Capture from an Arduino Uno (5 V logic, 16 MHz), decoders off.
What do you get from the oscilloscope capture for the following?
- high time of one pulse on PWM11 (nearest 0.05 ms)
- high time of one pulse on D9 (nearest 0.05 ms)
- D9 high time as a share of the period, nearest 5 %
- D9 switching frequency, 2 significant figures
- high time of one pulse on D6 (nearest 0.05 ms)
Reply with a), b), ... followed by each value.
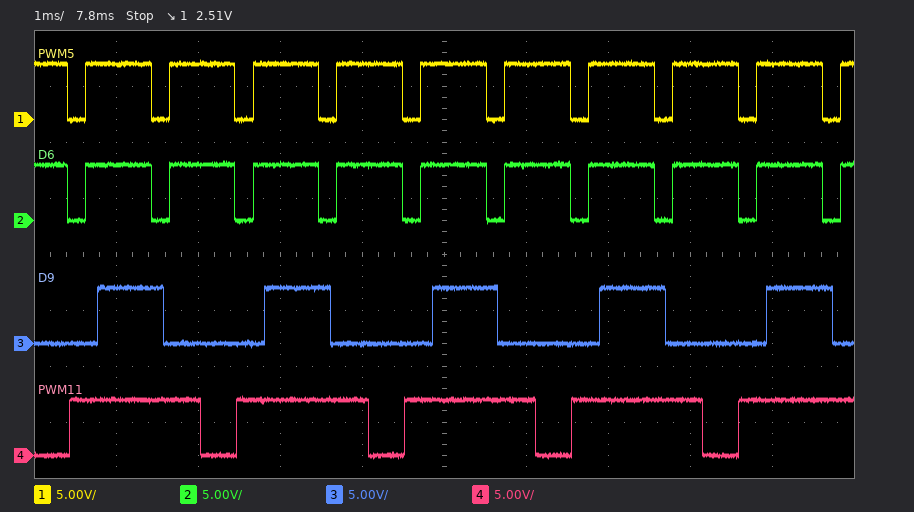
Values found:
a) 1.60 ms
b) 0.80 ms
c) 40 %
d) 490 Hz
e) 0.80 ms
